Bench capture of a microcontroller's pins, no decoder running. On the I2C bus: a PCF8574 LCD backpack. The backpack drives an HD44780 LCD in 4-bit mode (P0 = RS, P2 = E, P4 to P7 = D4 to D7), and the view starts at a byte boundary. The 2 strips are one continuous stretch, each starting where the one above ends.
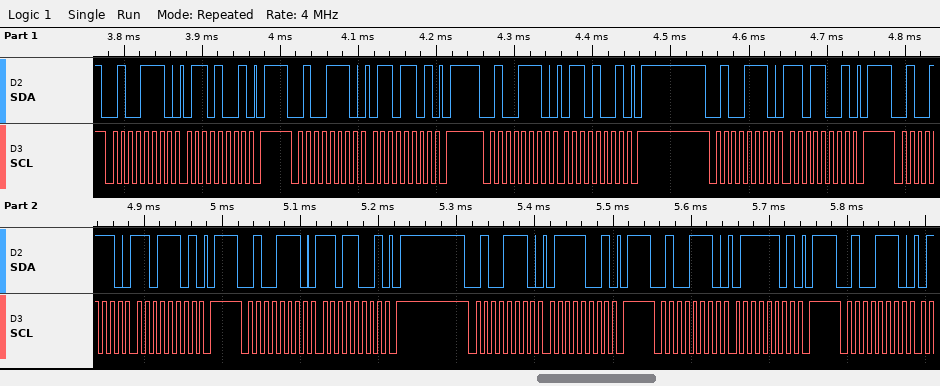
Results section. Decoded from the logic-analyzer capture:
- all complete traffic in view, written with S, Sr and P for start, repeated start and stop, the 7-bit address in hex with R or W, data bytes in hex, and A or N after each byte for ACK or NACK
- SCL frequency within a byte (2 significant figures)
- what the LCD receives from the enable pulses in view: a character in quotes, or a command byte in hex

S 27W A 69 A P S 27W A 6D A P S 27W A 69 A P S 27W A D9 A P S 27W A DD A P S 27W A D9 A P S 27W A 79 A P S 27W A 7D A P S 27W A
100 kHz
'm'
